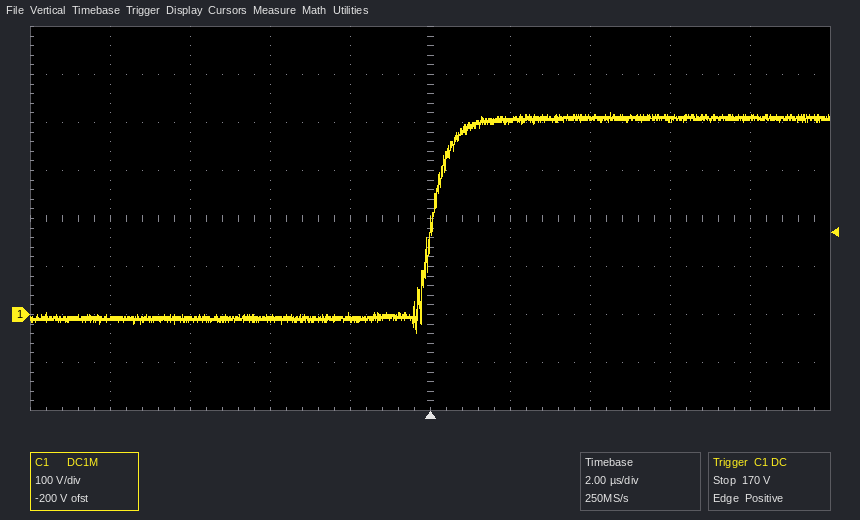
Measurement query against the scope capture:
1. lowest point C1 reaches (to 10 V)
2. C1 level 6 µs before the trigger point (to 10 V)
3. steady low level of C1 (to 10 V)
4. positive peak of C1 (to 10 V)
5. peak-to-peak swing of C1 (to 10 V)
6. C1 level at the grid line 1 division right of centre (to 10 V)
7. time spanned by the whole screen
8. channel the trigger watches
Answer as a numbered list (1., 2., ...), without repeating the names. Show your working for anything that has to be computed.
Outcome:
1. -40 V
2. -10 V
3. -10 V
4. 420 V
5. 420 V − (-40 V) = 460 V
6. 400 V
7. 20 µs
8. C1
